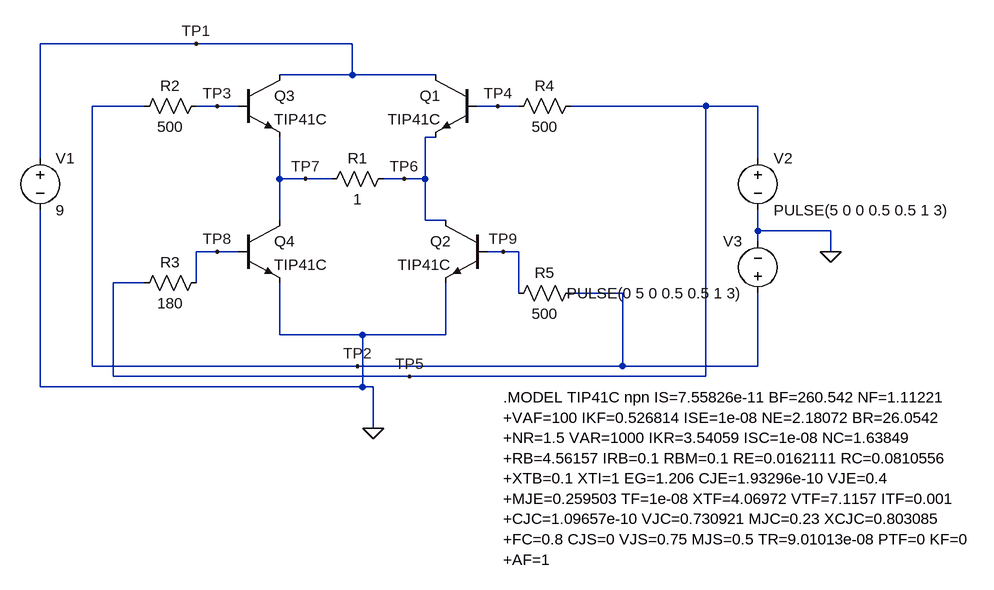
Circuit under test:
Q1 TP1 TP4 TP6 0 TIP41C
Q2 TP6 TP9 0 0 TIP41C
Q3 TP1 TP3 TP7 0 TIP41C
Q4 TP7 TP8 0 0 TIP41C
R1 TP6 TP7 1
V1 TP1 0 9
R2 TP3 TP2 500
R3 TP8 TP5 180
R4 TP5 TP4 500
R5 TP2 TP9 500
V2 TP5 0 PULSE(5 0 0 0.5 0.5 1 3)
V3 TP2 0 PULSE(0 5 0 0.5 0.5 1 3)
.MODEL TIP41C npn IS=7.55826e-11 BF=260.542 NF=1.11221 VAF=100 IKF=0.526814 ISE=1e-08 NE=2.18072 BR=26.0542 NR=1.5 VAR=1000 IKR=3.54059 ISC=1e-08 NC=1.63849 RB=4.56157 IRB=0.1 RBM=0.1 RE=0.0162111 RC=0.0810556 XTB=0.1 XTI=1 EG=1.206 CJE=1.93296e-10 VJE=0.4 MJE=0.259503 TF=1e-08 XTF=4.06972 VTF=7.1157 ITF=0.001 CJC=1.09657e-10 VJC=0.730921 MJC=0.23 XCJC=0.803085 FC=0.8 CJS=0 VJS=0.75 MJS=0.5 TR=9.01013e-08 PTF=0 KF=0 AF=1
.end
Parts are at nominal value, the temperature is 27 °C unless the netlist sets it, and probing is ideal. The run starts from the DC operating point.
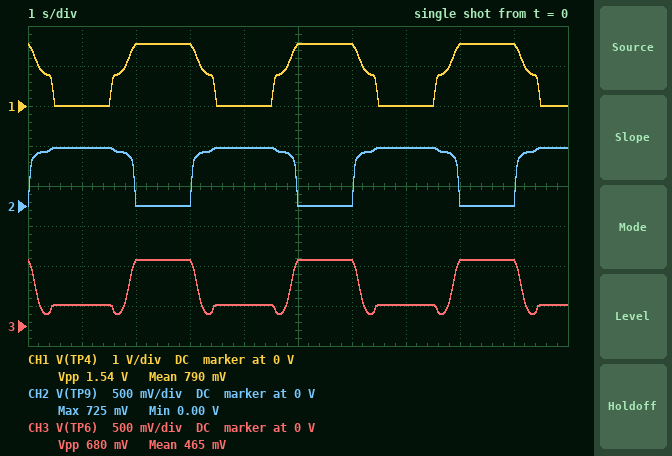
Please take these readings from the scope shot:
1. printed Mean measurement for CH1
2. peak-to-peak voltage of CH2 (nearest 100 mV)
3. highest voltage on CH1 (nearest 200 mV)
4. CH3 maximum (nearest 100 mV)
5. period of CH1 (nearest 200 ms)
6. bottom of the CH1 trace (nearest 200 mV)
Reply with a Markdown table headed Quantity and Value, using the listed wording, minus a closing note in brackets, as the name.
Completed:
| Quantity | Value |
|---|---|
| printed Mean measurement for CH1 | 790 mV |
| peak-to-peak voltage of CH2 | 700 mV |
| highest voltage on CH1 | 1.6 V |
| CH3 maximum | 800 mV |
| period of CH1 | 3.0 s |
| bottom of the CH1 trace | 0 V |
